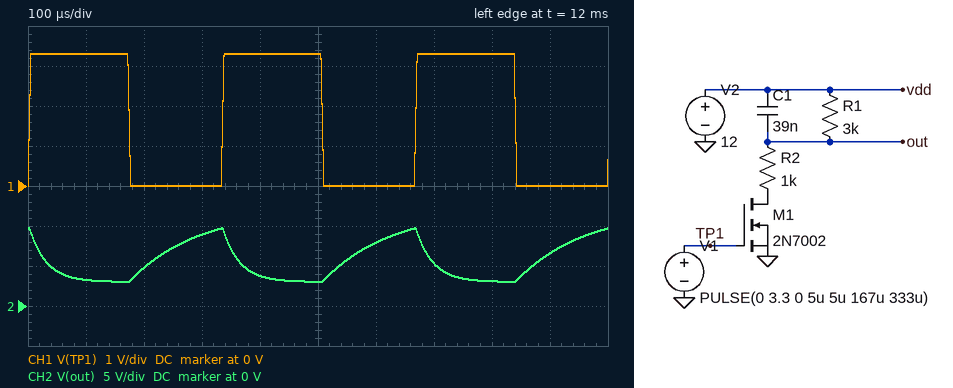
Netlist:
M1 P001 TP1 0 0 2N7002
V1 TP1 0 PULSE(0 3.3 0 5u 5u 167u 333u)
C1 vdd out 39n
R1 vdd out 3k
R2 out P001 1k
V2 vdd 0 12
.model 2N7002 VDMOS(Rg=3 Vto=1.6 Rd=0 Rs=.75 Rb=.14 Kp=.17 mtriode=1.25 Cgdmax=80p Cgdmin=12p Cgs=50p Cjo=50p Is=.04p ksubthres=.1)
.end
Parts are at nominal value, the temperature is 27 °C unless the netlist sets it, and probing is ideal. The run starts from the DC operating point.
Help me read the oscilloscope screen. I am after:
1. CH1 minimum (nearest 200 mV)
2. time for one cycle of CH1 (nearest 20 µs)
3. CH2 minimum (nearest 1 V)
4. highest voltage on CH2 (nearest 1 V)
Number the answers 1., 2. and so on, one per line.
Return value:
1. 0 V
2. 340 µs
3. 3 V
4. 10 V
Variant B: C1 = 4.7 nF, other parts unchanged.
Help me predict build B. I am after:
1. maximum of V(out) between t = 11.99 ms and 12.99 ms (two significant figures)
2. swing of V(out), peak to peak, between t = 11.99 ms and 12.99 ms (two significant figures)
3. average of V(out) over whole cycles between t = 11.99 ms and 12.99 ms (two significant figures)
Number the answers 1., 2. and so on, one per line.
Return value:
1. 12 V
2. 9.0 V
3. 7.1 V
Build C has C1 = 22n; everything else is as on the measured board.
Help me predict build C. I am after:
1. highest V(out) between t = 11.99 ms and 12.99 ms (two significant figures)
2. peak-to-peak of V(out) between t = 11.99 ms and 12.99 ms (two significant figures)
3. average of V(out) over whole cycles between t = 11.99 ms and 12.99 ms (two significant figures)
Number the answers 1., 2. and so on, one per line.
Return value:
1. 11 V
2. 8.2 V
3. 6.1 V
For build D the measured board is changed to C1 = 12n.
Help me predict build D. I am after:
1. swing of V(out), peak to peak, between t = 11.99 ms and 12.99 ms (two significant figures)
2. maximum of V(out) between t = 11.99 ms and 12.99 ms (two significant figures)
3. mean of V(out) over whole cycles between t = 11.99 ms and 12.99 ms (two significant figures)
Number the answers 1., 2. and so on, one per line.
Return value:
1. 8.9 V
2. 12 V
3. 6.6 V
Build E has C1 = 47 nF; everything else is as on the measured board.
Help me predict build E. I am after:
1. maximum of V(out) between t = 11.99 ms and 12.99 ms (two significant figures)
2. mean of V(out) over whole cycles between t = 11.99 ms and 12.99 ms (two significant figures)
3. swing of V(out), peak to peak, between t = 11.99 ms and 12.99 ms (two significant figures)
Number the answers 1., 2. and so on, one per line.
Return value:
1. 9.1 V
2. 5.4 V
3. 6.1 V
